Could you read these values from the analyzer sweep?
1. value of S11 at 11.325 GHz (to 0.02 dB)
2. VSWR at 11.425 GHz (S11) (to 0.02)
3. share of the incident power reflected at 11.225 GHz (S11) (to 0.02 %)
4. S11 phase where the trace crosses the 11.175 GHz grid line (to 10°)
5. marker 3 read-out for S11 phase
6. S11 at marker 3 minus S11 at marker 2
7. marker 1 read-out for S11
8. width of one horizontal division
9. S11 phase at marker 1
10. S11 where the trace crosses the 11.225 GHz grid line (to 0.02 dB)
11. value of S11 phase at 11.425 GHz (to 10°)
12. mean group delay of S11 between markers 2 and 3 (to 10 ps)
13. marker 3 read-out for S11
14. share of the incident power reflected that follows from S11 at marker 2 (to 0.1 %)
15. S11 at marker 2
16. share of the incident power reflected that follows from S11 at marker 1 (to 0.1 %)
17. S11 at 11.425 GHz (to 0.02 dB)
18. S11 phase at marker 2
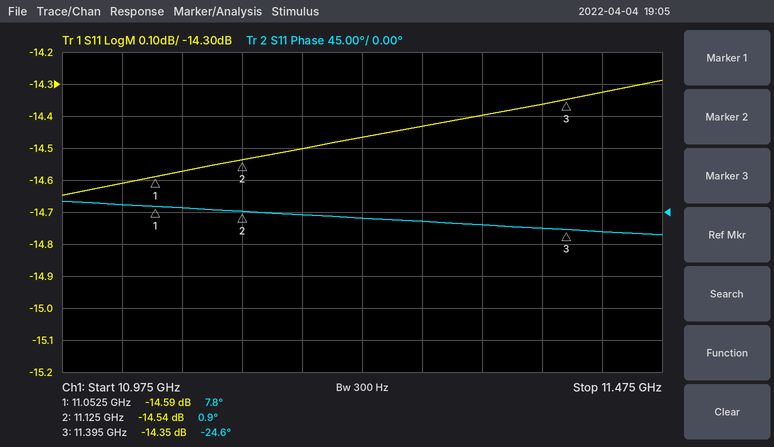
-14.40 dB
1.48
3.58 %
0°
-24.6°
0.19 dB
-14.59 dB
50 MHz
7.8°
-14.46 dB
-30°
260 ps
-14.35 dB
3.5 %
-14.54 dB
3.5 %
-14.32 dB
0.9°
